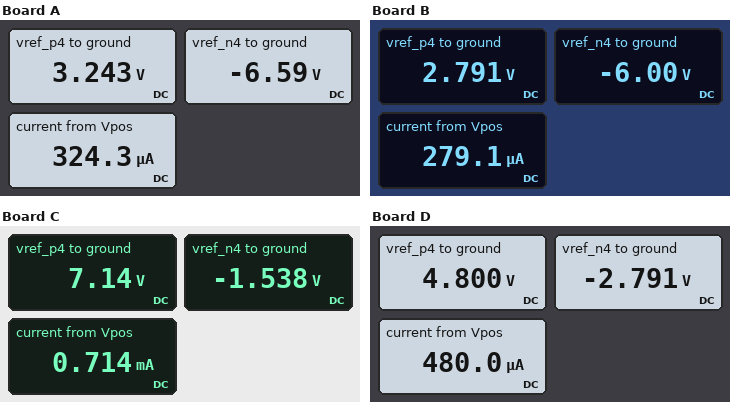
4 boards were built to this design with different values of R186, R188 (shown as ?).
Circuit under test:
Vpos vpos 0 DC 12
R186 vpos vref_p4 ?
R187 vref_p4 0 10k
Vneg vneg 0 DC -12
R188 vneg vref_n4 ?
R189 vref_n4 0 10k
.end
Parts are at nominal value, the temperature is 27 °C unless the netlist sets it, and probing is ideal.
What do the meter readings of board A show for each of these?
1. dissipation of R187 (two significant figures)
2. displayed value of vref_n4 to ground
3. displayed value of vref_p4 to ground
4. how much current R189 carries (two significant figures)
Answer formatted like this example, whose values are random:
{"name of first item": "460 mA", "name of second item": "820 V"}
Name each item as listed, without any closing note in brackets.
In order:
{"dissipation of R187": "1.1 mW", "displayed value of vref_n4 to ground": "-6.59 V", "displayed value of vref_p4 to ground": "3.243 V", "how much current R189 carries": "660 µA"}
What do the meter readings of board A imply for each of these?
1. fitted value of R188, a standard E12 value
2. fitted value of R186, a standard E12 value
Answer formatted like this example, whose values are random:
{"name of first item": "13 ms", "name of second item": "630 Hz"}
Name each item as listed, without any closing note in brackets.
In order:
{"fitted value of R188, a standard E12 value": "8.2 kΩ", "fitted value of R186, a standard E12 value": "27 kΩ"}
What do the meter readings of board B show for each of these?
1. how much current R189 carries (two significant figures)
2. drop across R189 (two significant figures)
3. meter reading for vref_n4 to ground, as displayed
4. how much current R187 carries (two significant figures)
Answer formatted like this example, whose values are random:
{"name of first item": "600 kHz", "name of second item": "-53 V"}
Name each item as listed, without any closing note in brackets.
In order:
{"how much current R189 carries": "600 µA", "drop across R189": "6.0 V", "meter reading for vref_n4 to ground, as displayed": "-6.00 V", "how much current R187 carries": "280 µA"}
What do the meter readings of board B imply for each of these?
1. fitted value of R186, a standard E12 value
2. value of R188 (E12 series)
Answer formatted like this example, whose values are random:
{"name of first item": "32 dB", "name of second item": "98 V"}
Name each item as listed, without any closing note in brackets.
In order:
{"fitted value of R186, a standard E12 value": "33 kΩ", "value of R188": "10 kΩ"}
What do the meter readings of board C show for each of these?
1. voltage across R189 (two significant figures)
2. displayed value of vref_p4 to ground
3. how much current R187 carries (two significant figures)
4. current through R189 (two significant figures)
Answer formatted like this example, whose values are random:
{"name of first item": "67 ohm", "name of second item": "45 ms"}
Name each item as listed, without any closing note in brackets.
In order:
{"voltage across R189": "1.5 V", "displayed value of vref_p4 to ground": "7.14 V", "how much current R187 carries": "710 µA", "current through R189": "150 µA"}
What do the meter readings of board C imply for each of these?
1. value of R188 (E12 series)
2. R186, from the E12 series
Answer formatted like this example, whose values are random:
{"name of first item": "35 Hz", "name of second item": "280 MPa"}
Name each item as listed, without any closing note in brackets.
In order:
{"value of R188": "68 kΩ", "R186, from the E12 series": "6.8 kΩ"}
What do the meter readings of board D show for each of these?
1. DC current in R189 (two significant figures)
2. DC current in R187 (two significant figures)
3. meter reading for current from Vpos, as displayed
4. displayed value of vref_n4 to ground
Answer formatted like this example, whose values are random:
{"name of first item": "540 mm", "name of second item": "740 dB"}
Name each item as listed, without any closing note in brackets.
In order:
{"DC current in R189": "280 µA", "DC current in R187": "480 µA", "meter reading for current from Vpos, as displayed": "480.0 µA", "displayed value of vref_n4 to ground": "-2.791 V"}
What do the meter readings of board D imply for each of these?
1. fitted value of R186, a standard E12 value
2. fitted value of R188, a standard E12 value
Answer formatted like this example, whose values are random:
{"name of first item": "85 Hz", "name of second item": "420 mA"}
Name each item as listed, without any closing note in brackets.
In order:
{"fitted value of R186, a standard E12 value": "15 kΩ", "fitted value of R188, a standard E12 value": "33 kΩ"}
